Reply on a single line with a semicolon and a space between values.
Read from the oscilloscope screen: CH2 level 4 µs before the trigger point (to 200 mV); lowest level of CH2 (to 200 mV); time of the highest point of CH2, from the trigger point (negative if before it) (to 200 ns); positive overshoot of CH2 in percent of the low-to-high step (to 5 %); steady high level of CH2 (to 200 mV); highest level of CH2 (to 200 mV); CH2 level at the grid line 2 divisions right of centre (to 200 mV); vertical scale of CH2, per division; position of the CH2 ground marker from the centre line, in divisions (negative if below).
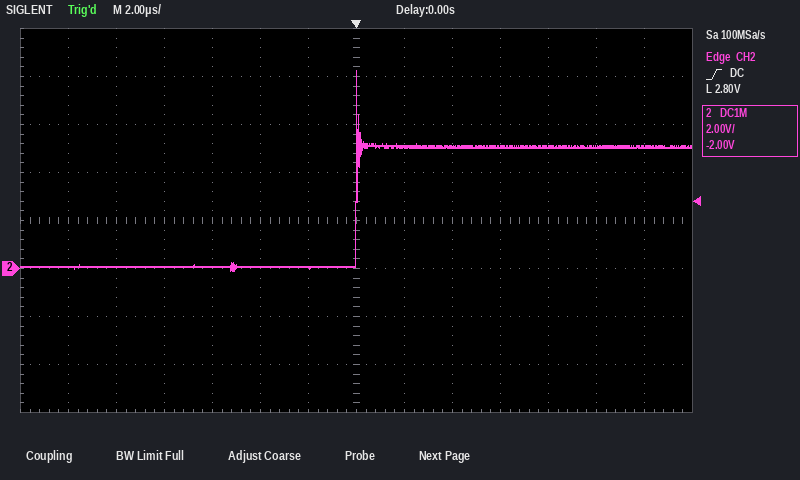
0.0 V; 0.0 V; 0.0 µs; 65 %; 5.0 V; 8.2 V; 5.0 V; 2 V; -1.0 div
